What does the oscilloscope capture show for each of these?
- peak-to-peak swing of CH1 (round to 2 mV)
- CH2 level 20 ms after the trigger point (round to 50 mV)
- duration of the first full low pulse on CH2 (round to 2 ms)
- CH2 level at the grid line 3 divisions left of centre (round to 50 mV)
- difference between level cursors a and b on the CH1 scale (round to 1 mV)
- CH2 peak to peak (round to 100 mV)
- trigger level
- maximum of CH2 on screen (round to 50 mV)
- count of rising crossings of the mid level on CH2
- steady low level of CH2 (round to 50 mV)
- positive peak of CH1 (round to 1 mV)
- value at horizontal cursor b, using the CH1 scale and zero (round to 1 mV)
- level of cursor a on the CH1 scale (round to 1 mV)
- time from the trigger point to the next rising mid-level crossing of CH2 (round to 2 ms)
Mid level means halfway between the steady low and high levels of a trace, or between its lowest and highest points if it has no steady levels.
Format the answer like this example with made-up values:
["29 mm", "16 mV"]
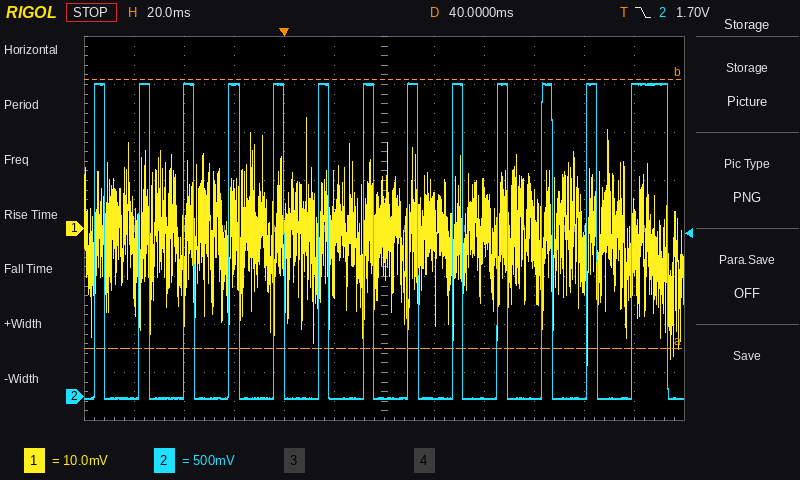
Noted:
["52 mV", "0 mV", "14 ms", "3.25 V", "56 mV", "3.30 V", "1.70 V", "3.25 V", "13", "0 mV", "23 mV", "31 mV", "-25 mV", "14 ms"]
